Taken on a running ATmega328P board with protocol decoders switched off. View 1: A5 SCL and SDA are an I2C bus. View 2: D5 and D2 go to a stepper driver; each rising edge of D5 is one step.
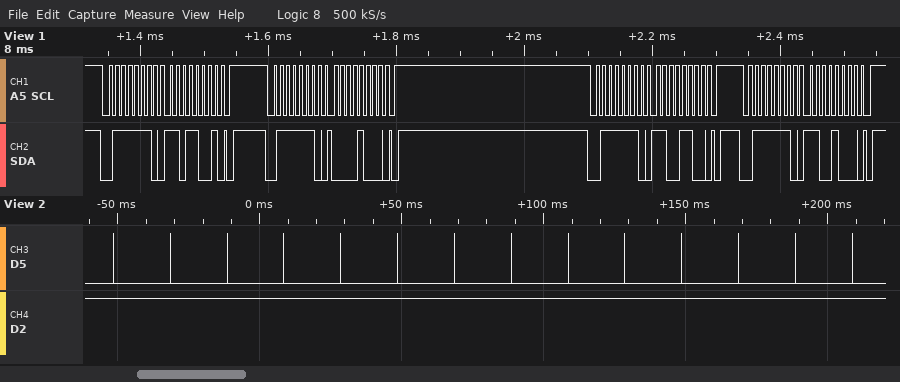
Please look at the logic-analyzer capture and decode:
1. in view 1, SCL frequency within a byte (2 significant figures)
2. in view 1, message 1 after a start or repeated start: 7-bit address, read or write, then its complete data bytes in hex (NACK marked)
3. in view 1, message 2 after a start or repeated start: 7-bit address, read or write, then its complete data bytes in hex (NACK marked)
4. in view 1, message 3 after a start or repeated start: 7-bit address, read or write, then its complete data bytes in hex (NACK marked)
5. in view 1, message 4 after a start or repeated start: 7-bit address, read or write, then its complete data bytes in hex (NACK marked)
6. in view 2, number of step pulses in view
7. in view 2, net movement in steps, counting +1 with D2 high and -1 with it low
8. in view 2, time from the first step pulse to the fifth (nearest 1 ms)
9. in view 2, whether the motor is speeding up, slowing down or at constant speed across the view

100 kHz
0x3F write: D9
0x3F write: 08
0x3F write: CC
0x3F write: C8
14
+14
80 ms
constant speed
